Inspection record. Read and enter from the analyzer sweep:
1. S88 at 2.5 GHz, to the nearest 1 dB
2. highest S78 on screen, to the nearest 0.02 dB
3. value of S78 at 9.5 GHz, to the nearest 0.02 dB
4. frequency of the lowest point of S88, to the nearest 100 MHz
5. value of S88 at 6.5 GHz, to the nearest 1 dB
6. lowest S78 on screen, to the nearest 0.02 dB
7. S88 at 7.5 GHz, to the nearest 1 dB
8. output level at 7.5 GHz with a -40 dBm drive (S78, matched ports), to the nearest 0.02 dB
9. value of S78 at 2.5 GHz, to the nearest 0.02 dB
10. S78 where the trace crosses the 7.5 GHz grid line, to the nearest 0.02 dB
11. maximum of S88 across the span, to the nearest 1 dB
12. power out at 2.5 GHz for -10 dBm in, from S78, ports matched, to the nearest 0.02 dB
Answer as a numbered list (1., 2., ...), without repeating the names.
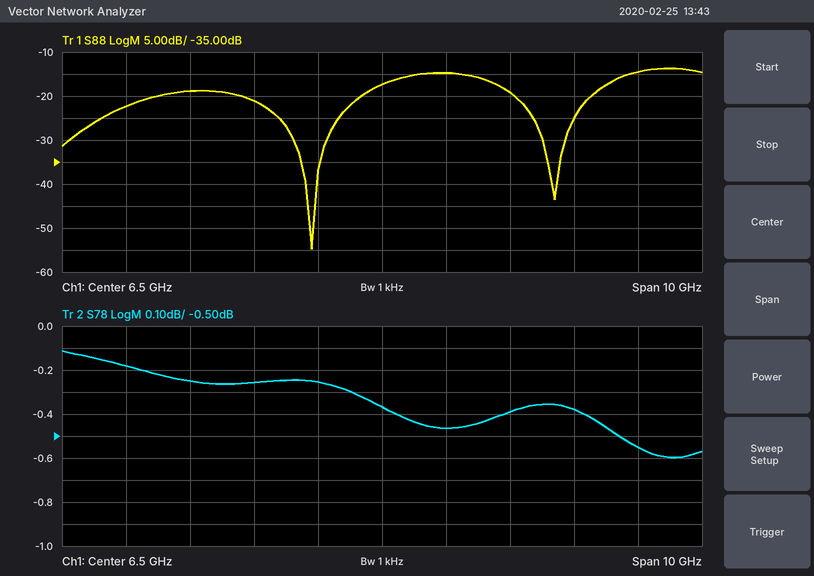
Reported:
1. -22 dB
2. -0.12 dB
3. -0.38 dB
4. 5.4 GHz
5. -17 dB
6. -0.60 dB
7. -15 dB
8. -40.46 dBm
9. -0.18 dB
10. -0.46 dB
11. -14 dB
12. -10.18 dBm
